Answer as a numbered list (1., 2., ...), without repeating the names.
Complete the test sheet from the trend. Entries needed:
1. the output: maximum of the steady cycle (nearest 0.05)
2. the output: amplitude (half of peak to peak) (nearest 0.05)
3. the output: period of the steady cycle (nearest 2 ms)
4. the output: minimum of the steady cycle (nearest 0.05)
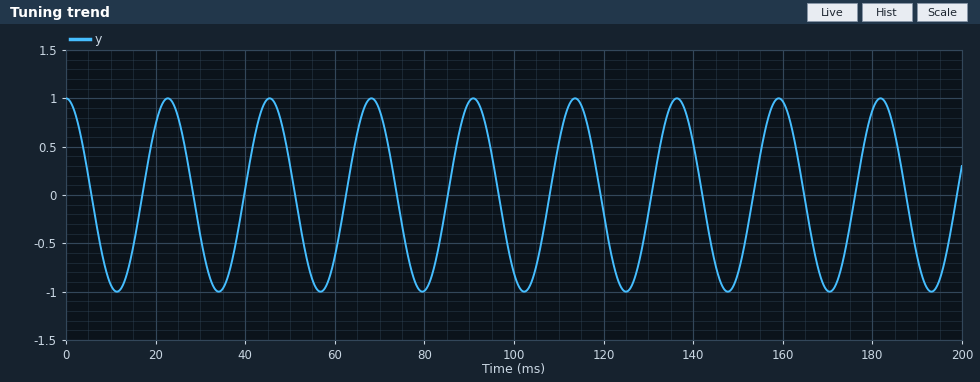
1. 1.00
2. 1.00
3. 22 ms
4. -1.00
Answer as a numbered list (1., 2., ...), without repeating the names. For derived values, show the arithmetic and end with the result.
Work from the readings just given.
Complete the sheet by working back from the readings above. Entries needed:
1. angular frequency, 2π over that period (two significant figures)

1. 2π / 22 = 0.29 rad/ms
